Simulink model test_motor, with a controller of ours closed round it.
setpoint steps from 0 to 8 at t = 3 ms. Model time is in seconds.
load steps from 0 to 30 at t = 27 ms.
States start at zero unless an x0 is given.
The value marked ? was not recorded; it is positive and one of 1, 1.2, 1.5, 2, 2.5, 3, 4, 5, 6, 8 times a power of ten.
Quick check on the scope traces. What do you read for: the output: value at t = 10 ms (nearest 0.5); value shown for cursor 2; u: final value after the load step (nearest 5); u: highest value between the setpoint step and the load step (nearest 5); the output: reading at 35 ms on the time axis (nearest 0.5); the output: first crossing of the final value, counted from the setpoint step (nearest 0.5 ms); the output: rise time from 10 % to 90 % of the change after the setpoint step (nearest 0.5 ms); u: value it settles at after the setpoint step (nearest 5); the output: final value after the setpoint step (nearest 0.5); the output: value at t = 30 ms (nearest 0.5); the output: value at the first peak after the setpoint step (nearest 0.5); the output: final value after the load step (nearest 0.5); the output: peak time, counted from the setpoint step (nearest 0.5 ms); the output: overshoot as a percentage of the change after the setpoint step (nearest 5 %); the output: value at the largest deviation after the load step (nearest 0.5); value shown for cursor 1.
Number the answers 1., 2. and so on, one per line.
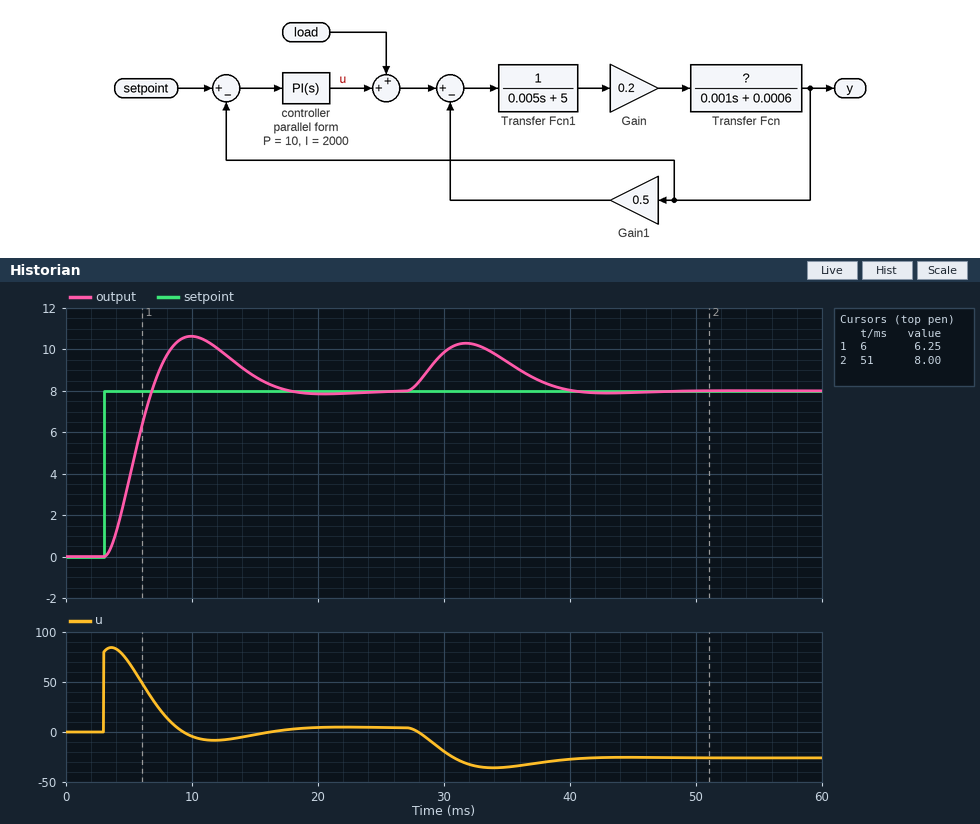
1. 10.5
2. 8.00
3. -25
4. 85
5. 9.5
6. 4.0 ms
7. 2.5 ms
8. 5
9. 8.0
10. 10.0
11. 10.5
12. 8.0
13. 7.0 ms
14. 35 %
15. 10.5
16. 6.25
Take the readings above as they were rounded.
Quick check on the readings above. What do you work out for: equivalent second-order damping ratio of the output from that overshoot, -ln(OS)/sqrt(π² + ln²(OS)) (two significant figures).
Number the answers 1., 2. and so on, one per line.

1. 0.32
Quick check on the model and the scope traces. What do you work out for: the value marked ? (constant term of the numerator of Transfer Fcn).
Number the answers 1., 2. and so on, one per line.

1. 1
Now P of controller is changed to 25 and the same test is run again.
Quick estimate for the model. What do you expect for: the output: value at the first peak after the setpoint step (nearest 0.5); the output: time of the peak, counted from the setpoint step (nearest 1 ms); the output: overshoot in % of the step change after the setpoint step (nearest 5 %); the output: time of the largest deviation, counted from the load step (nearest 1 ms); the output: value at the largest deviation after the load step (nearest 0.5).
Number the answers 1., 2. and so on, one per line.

1. 10.0
2. 4 ms
3. 25 %
4. 3 ms
5. 9.5
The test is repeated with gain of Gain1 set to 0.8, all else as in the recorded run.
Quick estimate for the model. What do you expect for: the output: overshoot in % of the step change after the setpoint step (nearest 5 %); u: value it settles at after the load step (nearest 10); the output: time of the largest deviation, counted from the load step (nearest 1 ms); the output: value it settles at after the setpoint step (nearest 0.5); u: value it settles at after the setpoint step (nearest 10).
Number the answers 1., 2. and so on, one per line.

1. 30 %
2. -20
3. 5 ms
4. 8.0
5. 10
